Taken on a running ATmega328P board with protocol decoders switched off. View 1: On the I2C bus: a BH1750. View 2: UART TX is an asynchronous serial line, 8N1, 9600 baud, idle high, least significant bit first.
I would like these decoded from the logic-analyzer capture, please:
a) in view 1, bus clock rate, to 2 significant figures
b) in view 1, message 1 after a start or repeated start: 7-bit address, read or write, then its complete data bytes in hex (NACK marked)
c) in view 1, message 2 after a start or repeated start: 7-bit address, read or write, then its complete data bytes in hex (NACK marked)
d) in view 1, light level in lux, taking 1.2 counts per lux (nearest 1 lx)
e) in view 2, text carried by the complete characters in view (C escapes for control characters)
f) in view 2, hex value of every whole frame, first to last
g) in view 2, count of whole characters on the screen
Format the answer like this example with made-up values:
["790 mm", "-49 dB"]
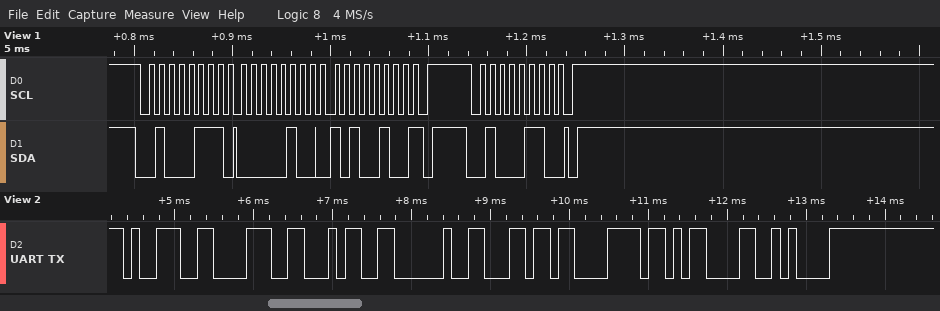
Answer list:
["100 kHz", "0x23 read: 04 A4 NACK", "0x23 write", "990 lx", "\"984 lx\\r\\n\"", "39 38 34 20 6C 78 0D 0A", "8"]
